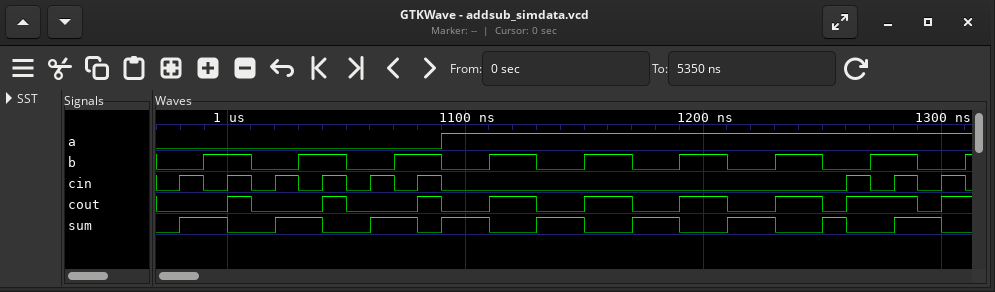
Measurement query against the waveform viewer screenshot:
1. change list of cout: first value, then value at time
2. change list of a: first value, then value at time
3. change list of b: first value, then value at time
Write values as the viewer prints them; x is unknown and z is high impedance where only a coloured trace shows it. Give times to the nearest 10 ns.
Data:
0, 1 at 1000 ns, 0 at 1010 ns, 1 at 1040 ns, 0 at 1050 ns, 1 at 1080 ns, 0 at 1090 ns, 1 at 1110 ns, 0 at 1130 ns, 1 at 1150 ns, 0 at 1170 ns, 1 at 1190 ns, 0 at 1210 ns, 1 at 1230 ns, 0 at 1250 ns, 1 at 1260 ns, 0 at 1290 ns, 1 at 1300 ns
0, 1 at 1090 ns
0, 1 at 990 ns, 0 at 1010 ns, 1 at 1030 ns, 0 at 1050 ns, 1 at 1070 ns, 0 at 1090 ns, 1 at 1110 ns, 0 at 1130 ns, 1 at 1150 ns, 0 at 1170 ns, 1 at 1190 ns, 0 at 1210 ns, 1 at 1230 ns, 0 at 1250 ns, 1 at 1270 ns, 0 at 1290 ns, 1 at 1310 ns
